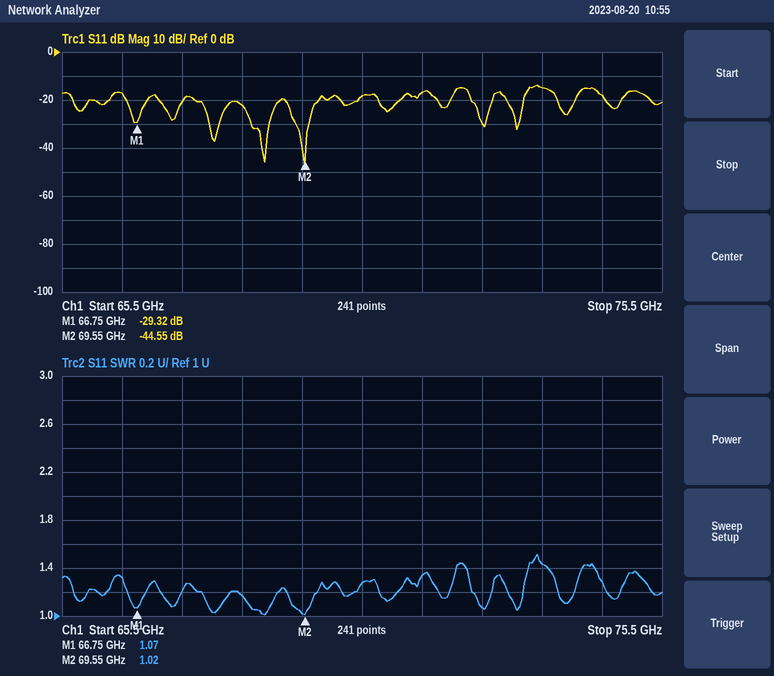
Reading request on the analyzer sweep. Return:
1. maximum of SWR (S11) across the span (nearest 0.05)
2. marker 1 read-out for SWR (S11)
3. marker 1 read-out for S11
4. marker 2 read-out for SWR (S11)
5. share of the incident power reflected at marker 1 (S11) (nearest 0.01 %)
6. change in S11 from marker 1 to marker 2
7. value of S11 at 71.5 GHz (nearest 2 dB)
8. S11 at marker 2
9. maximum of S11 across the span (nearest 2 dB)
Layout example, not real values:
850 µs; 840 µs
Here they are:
1.50; 1.07; -29.32 dB; 1.02; 0.12 %; -15.23 dB; -16 dB; -44.55 dB; -14 dB
